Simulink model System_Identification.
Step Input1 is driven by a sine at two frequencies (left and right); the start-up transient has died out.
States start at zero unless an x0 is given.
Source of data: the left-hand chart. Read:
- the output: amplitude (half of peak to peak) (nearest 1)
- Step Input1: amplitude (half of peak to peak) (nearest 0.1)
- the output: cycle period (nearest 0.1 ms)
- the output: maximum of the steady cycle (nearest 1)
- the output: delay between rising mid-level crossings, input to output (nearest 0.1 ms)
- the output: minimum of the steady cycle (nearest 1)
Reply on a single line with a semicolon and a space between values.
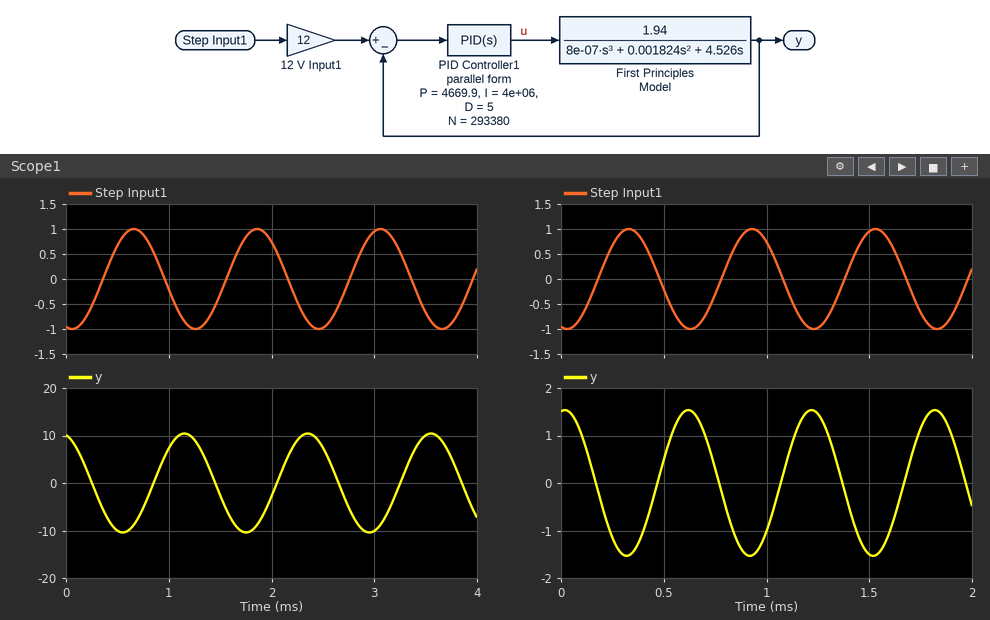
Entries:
10; 1.0; 1.2 ms; 10; 0.5 ms; -10
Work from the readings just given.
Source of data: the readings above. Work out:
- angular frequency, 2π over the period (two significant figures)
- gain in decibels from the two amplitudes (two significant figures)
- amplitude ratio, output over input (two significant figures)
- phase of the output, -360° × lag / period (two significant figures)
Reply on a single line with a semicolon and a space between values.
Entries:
5.2 rad/ms; 20 dB; 10; -150°
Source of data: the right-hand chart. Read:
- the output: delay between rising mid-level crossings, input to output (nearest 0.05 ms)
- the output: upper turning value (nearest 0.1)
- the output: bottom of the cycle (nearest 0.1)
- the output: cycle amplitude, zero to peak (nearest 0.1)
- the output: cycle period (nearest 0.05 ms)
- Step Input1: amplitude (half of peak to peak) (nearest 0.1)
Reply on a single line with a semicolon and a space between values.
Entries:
0.30 ms; 1.5; -1.5; 1.5; 0.60 ms; 1.0
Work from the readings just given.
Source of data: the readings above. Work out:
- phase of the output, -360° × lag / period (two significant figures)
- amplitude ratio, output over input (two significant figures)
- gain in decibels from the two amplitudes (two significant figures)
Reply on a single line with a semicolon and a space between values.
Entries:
-180°; 1.5; 3.5 dB
